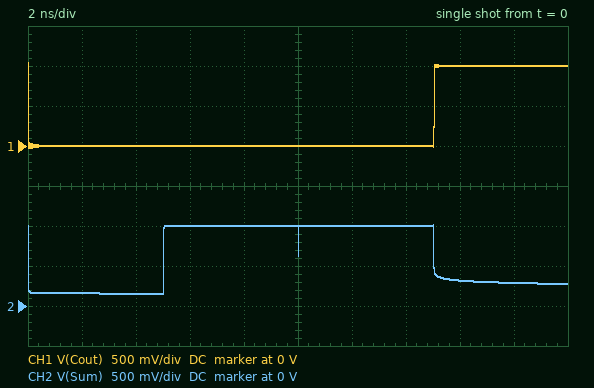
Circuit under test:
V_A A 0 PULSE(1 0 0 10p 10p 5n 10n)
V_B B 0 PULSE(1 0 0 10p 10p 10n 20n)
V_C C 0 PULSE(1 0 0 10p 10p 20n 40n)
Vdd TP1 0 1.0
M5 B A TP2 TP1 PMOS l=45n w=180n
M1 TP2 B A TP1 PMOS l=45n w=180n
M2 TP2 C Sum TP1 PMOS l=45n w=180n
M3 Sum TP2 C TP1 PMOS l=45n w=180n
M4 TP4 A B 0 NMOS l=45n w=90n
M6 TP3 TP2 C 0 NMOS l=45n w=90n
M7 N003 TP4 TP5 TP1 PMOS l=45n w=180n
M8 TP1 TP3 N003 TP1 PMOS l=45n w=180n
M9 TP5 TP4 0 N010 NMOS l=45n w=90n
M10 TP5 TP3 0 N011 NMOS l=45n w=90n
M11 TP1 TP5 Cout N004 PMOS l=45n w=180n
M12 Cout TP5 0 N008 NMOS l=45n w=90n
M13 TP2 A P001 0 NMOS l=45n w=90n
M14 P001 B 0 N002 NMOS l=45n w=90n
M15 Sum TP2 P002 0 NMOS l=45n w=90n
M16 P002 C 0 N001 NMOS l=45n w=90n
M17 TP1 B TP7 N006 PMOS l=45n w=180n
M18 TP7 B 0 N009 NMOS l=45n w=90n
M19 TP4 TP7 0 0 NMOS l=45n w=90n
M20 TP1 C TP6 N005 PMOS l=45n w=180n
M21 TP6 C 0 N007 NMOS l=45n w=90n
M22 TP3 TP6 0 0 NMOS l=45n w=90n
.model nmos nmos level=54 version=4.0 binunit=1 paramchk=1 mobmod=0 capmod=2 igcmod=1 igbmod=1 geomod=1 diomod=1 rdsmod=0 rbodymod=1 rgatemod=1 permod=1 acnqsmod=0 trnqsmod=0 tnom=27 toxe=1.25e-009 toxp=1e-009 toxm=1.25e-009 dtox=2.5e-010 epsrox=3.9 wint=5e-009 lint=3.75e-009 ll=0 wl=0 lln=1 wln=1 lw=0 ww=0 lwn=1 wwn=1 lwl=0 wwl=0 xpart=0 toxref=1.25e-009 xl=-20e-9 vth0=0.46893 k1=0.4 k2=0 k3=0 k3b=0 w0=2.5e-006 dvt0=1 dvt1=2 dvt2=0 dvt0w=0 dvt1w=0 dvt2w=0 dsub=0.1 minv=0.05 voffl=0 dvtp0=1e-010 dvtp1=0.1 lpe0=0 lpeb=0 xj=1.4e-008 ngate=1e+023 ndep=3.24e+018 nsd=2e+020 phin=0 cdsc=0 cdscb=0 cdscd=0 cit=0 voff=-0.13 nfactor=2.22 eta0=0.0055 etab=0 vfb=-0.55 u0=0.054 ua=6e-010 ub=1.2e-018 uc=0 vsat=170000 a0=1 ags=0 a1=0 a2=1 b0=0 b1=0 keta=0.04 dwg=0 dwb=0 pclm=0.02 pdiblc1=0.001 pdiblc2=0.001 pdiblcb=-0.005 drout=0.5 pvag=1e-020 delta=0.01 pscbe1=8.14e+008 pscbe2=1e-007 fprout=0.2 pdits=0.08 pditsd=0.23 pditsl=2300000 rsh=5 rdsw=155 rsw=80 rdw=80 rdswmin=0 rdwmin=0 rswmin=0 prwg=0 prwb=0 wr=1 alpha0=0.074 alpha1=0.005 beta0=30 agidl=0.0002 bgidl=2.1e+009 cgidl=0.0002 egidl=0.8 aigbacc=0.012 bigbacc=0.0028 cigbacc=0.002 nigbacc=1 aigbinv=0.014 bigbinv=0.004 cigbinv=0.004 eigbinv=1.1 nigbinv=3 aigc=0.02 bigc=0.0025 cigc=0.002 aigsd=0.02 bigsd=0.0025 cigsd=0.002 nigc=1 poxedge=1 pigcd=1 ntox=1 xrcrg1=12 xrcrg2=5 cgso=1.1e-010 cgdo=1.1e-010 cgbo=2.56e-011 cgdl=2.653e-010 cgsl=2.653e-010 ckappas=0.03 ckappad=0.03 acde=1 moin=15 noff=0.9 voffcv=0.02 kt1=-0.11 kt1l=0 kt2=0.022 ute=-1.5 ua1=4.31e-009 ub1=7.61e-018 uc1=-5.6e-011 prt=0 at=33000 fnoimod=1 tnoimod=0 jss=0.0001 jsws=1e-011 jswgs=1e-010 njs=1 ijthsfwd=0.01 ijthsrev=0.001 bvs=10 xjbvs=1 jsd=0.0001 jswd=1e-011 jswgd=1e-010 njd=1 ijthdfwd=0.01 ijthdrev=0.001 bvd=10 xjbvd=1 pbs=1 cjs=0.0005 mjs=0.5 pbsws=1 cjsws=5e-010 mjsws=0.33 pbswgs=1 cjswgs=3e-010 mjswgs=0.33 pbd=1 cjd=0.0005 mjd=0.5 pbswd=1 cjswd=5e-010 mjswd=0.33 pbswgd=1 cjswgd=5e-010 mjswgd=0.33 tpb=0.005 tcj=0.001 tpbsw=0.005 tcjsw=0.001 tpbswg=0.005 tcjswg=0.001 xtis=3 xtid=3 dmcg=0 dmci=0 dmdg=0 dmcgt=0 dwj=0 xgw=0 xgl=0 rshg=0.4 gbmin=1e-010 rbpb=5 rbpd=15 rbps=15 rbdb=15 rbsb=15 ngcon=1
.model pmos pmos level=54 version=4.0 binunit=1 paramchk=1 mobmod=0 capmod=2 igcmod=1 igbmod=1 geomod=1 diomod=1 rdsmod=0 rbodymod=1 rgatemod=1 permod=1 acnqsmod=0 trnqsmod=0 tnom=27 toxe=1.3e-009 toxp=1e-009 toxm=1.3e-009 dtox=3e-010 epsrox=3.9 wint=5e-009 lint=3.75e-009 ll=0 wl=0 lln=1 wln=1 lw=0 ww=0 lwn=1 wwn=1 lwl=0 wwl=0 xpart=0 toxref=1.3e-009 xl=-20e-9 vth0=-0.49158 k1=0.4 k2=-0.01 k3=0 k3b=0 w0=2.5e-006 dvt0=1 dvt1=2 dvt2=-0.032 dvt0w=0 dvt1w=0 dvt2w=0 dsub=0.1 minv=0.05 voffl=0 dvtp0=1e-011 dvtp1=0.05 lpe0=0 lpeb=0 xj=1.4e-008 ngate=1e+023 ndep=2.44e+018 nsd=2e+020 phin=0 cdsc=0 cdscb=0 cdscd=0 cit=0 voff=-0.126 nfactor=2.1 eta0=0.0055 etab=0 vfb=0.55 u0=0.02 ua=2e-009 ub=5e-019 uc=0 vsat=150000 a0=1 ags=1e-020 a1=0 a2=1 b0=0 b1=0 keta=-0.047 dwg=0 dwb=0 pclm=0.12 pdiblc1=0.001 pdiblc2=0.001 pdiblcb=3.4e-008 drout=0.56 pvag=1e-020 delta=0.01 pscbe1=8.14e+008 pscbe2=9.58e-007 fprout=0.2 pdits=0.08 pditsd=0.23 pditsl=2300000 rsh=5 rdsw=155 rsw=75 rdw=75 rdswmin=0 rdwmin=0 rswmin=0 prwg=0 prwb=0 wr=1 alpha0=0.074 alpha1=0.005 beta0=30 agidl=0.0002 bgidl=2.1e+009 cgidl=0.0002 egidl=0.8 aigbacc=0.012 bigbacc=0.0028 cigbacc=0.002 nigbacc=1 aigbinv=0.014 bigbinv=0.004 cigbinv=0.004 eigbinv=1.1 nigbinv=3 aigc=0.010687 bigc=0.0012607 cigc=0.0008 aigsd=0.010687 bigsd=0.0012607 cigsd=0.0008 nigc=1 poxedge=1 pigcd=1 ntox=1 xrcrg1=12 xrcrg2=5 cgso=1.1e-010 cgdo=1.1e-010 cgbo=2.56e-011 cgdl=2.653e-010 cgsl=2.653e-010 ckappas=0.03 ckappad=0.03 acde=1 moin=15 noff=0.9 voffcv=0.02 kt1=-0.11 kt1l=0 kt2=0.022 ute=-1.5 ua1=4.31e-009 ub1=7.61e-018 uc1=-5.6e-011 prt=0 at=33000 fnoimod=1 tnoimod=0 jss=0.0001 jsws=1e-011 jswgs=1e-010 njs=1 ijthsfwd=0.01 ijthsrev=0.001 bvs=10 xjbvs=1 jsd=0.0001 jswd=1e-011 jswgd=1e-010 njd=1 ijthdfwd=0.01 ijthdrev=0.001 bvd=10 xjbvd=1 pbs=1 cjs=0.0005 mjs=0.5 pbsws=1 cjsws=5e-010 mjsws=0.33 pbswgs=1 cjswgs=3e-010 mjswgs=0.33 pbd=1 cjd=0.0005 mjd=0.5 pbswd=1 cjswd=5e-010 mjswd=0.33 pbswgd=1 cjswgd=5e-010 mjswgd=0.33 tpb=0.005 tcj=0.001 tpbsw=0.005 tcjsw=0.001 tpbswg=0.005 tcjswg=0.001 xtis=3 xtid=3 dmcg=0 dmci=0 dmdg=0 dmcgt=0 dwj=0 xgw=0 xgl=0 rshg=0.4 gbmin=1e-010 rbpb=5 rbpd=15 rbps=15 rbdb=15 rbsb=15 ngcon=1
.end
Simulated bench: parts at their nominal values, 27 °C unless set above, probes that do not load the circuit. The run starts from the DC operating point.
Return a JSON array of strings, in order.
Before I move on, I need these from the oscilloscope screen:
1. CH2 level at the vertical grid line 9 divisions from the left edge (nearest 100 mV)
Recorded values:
["300 mV"]
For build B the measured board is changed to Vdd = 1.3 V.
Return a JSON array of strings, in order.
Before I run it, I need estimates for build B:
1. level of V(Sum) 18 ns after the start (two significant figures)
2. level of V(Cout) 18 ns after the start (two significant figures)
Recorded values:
["320 mV", "1.3 V"]
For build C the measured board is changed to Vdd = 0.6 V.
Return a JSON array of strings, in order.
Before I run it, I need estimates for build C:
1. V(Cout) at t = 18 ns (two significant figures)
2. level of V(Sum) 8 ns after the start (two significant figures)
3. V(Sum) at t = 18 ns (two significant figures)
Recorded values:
["600 mV", "1.0 V", "240 mV"]
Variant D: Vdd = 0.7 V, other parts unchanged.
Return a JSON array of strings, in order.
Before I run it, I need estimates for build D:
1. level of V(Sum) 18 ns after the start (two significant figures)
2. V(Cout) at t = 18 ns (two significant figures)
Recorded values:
["250 mV", "700 mV"]
